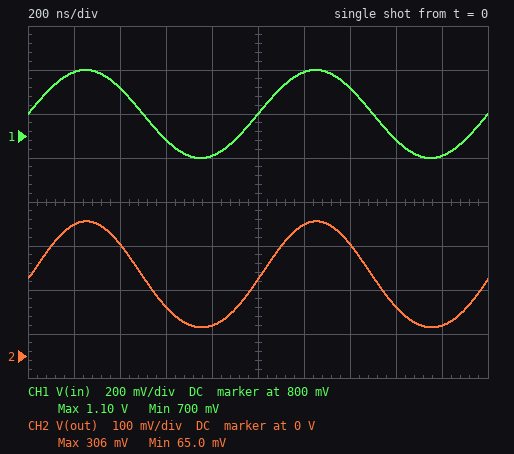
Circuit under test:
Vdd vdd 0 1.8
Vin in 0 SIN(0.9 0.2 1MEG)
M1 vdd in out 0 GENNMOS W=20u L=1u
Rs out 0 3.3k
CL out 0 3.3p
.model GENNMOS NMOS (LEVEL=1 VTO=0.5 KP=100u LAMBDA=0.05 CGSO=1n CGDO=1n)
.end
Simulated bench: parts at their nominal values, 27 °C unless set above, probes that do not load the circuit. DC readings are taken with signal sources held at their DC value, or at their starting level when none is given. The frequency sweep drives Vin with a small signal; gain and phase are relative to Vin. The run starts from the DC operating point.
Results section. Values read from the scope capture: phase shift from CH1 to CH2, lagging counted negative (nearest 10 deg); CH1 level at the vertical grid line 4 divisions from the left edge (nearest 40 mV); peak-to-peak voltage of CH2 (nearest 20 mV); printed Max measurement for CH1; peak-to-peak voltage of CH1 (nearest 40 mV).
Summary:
0 deg
720 mV
240 mV
1.10 V
400 mV
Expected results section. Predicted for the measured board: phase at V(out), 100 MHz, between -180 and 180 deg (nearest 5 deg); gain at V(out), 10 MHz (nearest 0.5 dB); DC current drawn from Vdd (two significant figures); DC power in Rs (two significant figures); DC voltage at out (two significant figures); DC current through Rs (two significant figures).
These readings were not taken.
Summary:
-70 deg
-4.5 dB
54 µA
9.5 µW
180 mV
54 µA
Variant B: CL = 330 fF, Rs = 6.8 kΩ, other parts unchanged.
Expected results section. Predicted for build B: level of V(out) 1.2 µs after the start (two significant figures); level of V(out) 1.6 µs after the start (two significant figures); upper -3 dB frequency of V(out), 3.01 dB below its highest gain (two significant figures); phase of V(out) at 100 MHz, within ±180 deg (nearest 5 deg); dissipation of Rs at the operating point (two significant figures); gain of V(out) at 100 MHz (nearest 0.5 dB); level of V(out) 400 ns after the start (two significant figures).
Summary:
370 mV
140 mV
240 MHz
-20 deg
7.4 µW
-3.5 dB
310 mV
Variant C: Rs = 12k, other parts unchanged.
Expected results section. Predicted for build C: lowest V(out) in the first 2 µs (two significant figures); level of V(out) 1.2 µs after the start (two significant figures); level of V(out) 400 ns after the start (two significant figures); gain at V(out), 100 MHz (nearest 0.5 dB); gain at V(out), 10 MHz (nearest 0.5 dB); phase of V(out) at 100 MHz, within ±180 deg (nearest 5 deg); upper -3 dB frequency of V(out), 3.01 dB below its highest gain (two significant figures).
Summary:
110 mV
410 mV
360 mV
-17.0 dB
-3.0 dB
-75 deg
19 MHz
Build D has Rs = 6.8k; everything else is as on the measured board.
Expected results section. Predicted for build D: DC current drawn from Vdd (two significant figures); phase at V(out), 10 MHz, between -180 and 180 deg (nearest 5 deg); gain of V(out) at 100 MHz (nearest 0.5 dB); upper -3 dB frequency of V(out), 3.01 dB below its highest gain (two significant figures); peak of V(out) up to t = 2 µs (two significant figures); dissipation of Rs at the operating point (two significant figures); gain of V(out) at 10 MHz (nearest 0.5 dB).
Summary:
33 µA
-20 deg
-15.0 dB
25 MHz
370 mV
7.4 µW
-3.5 dB
